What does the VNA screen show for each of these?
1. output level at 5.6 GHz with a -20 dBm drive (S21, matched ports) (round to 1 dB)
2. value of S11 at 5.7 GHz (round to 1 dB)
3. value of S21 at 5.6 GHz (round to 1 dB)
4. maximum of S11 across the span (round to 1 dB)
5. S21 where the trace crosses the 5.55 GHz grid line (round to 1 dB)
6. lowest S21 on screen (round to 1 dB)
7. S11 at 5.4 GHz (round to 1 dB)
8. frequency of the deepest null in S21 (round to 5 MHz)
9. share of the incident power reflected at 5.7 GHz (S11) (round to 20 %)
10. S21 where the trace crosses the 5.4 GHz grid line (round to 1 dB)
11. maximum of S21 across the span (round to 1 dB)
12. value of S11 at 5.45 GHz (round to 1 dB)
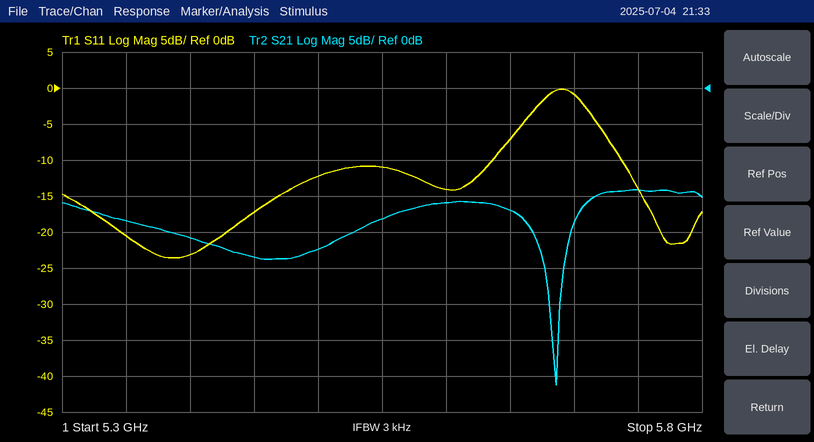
-36 dBm
-1 dB
-16 dB
0 dB
-18 dB
-41 dB
-23 dB
5.685 GHz
80 %
-21 dB
-14 dB
-17 dB
